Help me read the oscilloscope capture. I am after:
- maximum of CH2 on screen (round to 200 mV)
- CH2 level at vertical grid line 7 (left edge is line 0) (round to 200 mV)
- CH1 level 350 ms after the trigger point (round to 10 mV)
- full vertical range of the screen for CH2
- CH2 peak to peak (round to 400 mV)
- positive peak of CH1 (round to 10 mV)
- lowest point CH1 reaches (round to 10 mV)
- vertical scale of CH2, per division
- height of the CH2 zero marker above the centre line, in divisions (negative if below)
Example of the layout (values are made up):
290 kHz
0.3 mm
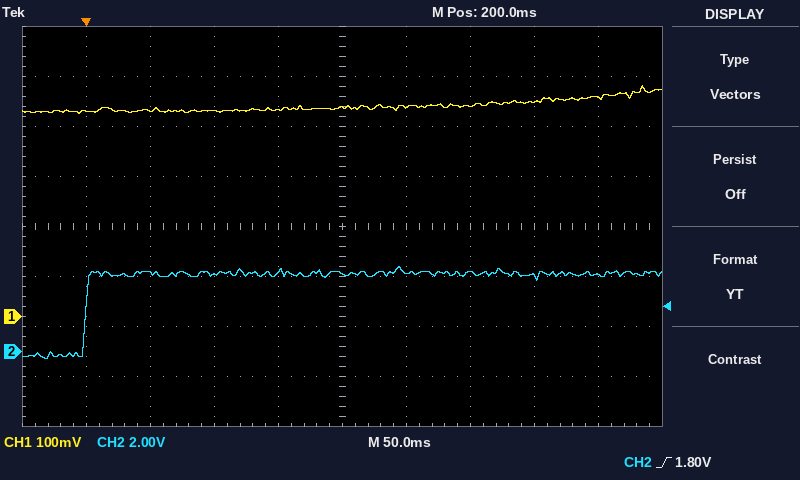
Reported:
3.4 V
3.2 V
430 mV
16 V
3.6 V
460 mV
410 mV
2 V
-2.5 div
